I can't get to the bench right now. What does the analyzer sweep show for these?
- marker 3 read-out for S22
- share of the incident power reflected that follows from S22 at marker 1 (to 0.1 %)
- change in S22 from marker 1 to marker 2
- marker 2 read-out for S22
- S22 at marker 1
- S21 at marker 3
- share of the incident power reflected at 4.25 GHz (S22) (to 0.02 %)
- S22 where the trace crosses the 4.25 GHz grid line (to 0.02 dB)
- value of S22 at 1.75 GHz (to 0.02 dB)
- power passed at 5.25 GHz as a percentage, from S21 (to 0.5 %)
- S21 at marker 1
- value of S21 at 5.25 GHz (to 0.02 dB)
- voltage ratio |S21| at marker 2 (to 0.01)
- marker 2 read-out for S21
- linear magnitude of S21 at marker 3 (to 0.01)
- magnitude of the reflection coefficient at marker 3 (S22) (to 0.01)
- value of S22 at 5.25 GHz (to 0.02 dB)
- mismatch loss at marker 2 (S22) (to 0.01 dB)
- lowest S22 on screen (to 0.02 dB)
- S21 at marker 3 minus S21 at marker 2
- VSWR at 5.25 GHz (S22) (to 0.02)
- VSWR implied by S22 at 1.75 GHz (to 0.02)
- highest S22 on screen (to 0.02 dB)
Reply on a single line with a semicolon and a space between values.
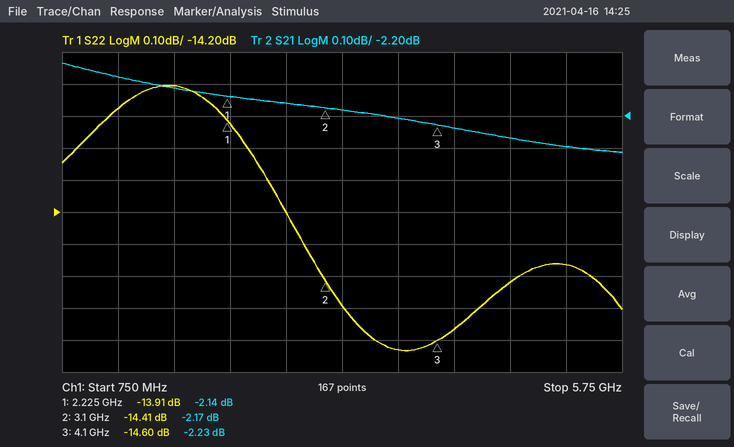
-14.60 dB; 4.1 %; -0.50 dB; -14.41 dB; -13.91 dB; -2.23 dB; 3.50 %; -14.56 dB; -13.80 dB; 59.0 %; -2.14 dB; -2.30 dB; 0.78; -2.17 dB; 0.77; 0.19; -14.36 dB; 0.16 dB; -14.64 dB; -0.06 dB; 1.48; 1.52; -13.80 dB
